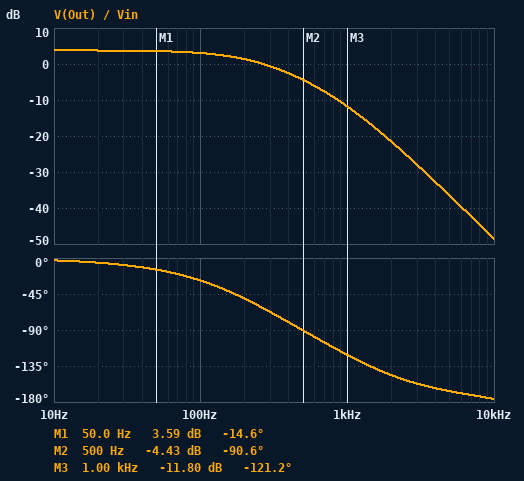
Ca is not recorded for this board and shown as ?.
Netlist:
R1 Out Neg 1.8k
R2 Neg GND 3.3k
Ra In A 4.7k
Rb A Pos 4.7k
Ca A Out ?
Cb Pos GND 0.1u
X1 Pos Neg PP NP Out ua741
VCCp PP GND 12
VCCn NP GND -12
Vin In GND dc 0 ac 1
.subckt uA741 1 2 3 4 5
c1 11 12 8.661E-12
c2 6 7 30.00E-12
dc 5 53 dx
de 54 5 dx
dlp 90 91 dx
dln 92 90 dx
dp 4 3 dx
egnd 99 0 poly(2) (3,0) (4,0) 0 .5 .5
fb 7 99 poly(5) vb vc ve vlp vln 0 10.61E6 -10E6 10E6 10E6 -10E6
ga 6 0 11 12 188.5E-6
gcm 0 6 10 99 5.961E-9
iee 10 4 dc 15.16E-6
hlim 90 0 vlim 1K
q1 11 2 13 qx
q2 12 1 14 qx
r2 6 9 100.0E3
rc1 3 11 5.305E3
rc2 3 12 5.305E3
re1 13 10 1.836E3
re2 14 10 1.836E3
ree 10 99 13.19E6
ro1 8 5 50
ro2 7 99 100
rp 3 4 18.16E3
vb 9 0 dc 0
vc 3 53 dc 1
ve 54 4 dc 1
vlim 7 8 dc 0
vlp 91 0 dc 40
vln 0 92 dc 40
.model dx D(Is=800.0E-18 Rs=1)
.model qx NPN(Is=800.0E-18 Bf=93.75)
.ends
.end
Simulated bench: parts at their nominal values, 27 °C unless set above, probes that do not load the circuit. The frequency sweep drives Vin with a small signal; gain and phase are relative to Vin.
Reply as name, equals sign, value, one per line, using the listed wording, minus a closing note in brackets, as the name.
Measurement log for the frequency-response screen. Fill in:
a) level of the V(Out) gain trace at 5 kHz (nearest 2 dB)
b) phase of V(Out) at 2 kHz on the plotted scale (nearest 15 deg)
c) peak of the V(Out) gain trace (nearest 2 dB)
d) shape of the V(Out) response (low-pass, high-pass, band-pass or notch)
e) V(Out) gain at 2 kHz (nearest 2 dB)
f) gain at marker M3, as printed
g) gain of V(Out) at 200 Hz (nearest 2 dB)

level of the V(Out) gain trace at 5 kHz = -36 dB
phase of V(Out) at 2 kHz on the plotted scale = -150 deg
peak of the V(Out) gain trace = 4 dB
shape of the V(Out) response = low-pass
V(Out) gain at 2 kHz = -22 dB
gain at marker M3, as printed = -11.80 dB
gain of V(Out) at 200 Hz = 2 dB
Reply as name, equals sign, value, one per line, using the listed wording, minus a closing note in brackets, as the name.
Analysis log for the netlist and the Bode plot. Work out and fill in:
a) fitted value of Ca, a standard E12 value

fitted value of Ca, a standard E12 value = 47 nF
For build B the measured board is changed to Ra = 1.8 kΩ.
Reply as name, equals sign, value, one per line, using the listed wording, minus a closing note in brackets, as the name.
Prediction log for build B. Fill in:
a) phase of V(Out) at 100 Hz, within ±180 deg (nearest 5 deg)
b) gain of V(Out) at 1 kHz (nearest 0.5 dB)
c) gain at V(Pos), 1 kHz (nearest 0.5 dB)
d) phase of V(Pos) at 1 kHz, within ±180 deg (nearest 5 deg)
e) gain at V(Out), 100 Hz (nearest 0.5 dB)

phase of V(Out) at 100 Hz, within ±180 deg = -20 deg
gain of V(Out) at 1 kHz = -8.0 dB
gain at V(Pos), 1 kHz = -11.5 dB
phase of V(Pos) at 1 kHz, within ±180 deg = -100 deg
gain at V(Out), 100 Hz = 3.5 dB
